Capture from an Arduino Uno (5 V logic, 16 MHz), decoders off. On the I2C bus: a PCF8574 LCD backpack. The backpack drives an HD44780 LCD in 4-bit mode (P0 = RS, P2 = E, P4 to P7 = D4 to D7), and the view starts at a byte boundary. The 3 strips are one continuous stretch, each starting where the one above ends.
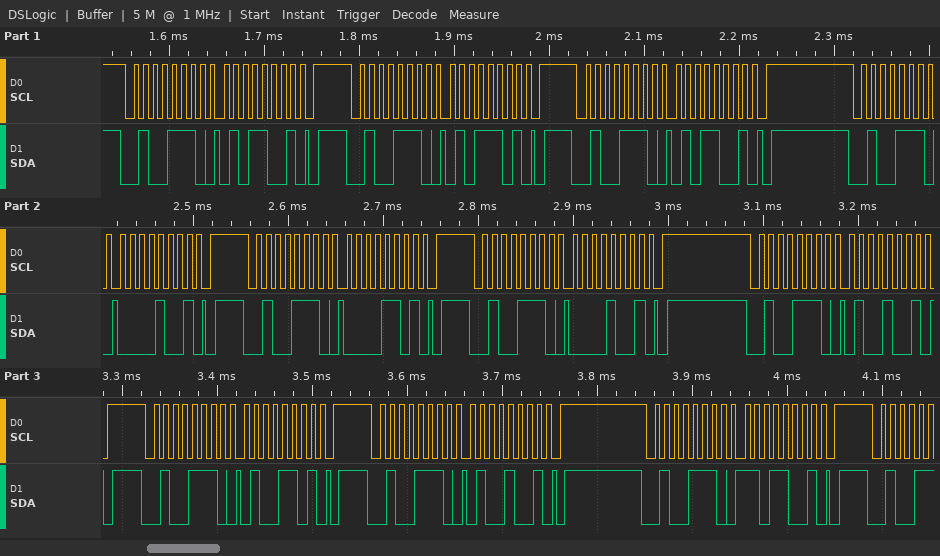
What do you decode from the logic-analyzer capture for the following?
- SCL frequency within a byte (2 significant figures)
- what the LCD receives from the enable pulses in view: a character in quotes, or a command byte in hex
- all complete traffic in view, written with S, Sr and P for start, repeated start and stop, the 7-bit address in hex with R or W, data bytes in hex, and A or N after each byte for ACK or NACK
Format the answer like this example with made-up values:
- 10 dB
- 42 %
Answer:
- 100 kHz
- 'P'
- S 27W A 59 A P S 27W A 5D A P S 27W A 59 A P S 27W A 09 A P S 27W A 0D A P S 27W A 09 A P S 27W A 49 A P S 27W A 4D A P S 27W A 49 A P S 27W A D9 A P
